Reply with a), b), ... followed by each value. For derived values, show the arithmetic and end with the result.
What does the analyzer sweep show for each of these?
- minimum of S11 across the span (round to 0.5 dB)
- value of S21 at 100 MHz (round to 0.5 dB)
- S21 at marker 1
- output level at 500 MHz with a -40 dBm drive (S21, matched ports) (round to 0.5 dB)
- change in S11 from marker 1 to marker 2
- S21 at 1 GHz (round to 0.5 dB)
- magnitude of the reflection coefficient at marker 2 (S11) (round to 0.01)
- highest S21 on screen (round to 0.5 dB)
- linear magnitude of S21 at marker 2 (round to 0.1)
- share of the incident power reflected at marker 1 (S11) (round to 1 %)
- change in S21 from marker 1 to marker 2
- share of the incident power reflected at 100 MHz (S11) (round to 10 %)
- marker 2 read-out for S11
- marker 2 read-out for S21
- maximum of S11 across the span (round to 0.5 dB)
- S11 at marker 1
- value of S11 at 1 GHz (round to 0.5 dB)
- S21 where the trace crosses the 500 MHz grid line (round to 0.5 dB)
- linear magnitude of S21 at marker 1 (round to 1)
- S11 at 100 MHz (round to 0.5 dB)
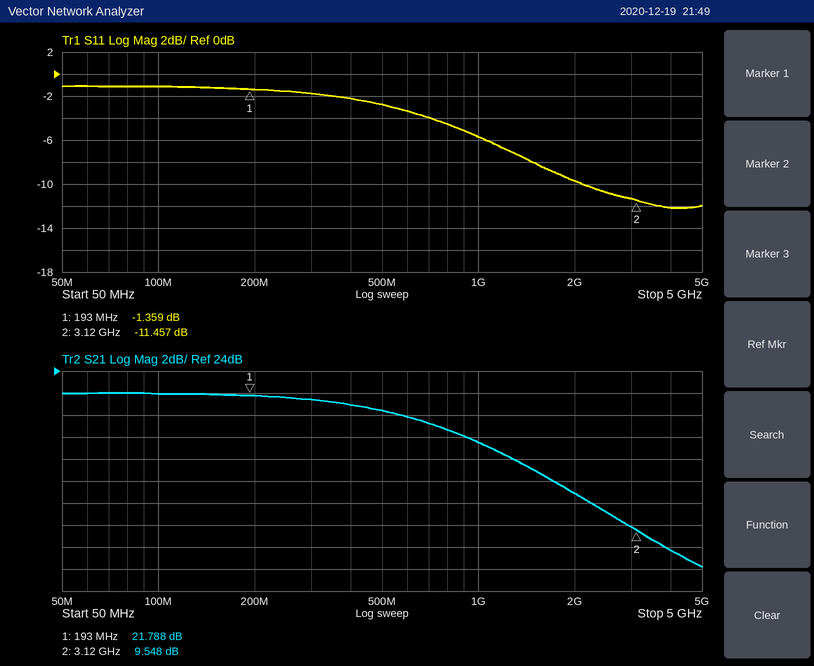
a) -12.0 dB
b) 22.0 dB
c) 21.788 dB
d) -40 dBm + (20.5 dB) = -19.5 dBm
e) -11.457 − (-1.359) = -10.098 dB
f) 17.5 dB
g) 10^(-11.457/20) ≈ 0.27
h) 22.0 dB
i) 10^(9.548/20) ≈ 3.0
j) 10^(-1.359/10) ≈ 73 %
k) 9.548 − (21.788) = -12.240 dB
l) 10^(-1/10) ≈ 79.4 %, so 80 % to the nearest 10 %
m) -11.457 dB
n) 9.548 dB
o) -1.0 dB
p) -1.359 dB
q) -5.5 dB
r) 20.5 dB
s) 10^(21.788/20) ≈ 12
t) -1.0 dB
